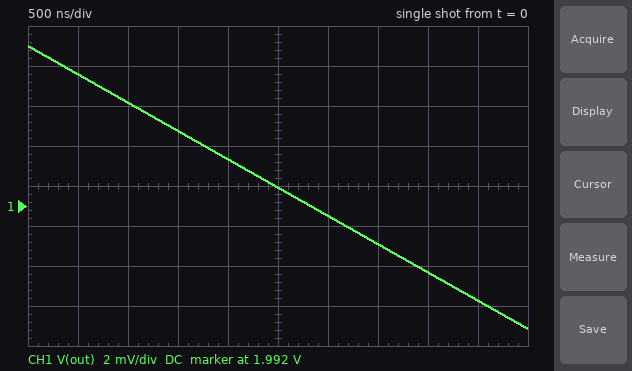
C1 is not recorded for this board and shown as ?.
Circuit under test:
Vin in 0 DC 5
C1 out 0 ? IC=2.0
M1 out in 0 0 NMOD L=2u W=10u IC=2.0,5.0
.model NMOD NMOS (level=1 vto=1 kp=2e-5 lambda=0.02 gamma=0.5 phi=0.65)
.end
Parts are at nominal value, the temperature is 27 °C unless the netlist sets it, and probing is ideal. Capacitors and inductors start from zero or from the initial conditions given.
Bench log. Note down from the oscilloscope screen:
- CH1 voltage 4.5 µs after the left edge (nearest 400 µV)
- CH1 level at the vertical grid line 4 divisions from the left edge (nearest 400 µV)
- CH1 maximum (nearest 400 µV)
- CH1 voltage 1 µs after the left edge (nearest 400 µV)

1.9872 V
1.9944 V
2.0000 V
1.9972 V
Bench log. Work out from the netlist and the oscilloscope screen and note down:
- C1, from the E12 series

220 nF
